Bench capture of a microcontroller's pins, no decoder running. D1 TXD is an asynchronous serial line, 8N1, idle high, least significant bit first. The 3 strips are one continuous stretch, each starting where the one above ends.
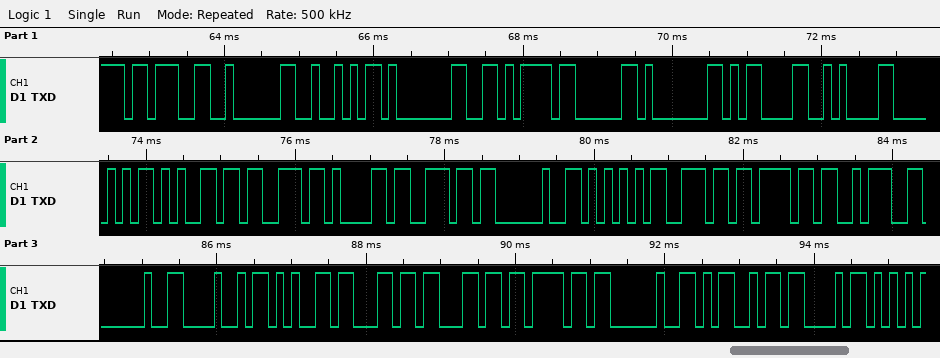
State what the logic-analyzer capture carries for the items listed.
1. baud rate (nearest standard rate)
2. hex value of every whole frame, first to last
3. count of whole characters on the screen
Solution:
9600 baud
3B 02 52 01 D6 03 01 0D 0A 50 65 73 61 6E 20 55 6E 6F 3A 20 48 65 6C 6C 6F 20 4D 43
28
